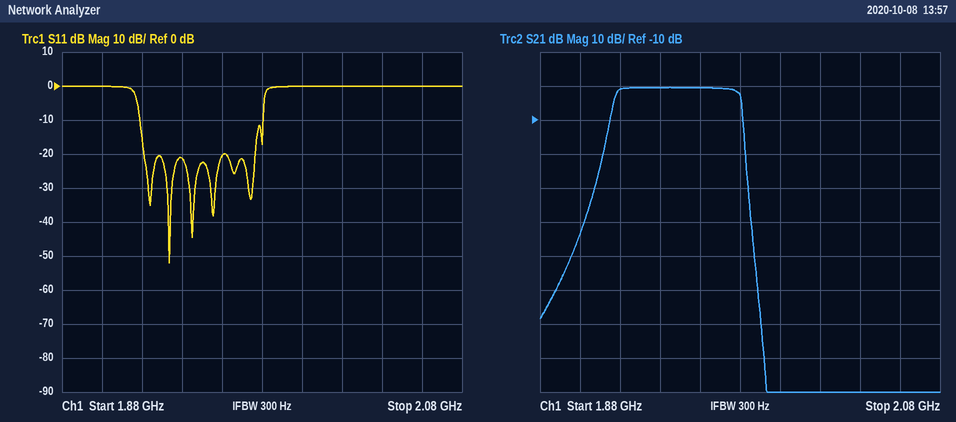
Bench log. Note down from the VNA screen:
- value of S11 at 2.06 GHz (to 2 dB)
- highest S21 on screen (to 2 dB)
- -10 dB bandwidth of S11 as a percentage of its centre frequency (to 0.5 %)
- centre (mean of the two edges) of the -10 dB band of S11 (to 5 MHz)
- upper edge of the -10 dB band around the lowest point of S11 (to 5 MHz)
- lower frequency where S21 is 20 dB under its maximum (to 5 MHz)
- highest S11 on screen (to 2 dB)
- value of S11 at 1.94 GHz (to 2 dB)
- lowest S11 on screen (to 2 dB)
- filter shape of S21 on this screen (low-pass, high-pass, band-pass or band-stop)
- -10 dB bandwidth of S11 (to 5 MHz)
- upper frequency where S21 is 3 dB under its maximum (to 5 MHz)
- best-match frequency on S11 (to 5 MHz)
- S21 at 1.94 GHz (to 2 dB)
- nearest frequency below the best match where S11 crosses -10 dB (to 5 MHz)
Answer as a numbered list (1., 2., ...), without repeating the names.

1. 0 dB
2. 0 dB
3. 3.0 %
4. 1.950 GHz
5. 1.980 GHz
6. 1.910 GHz
7. 0 dB
8. -22 dB
9. -52 dB
10. band-pass
11. 60 MHz
12. 1.980 GHz
13. 1.935 GHz
14. 0 dB
15. 1.920 GHz
